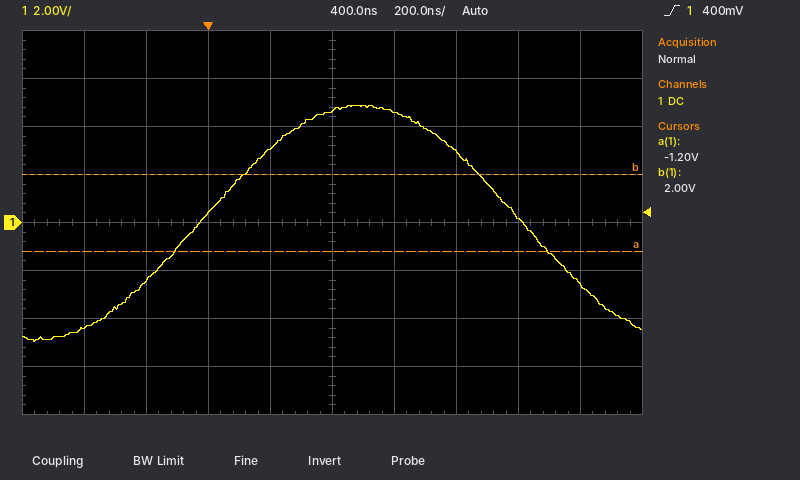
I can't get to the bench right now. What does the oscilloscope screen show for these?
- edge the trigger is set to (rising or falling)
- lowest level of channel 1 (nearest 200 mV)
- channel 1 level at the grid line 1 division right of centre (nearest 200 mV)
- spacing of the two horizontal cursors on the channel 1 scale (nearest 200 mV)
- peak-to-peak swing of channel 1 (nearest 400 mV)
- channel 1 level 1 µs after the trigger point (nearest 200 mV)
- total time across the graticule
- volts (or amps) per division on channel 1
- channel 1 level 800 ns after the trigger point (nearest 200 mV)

rising
-5.0 V
4.6 V
3.2 V
10.0 V
200 mV
2 µs
2 V
3.0 V
